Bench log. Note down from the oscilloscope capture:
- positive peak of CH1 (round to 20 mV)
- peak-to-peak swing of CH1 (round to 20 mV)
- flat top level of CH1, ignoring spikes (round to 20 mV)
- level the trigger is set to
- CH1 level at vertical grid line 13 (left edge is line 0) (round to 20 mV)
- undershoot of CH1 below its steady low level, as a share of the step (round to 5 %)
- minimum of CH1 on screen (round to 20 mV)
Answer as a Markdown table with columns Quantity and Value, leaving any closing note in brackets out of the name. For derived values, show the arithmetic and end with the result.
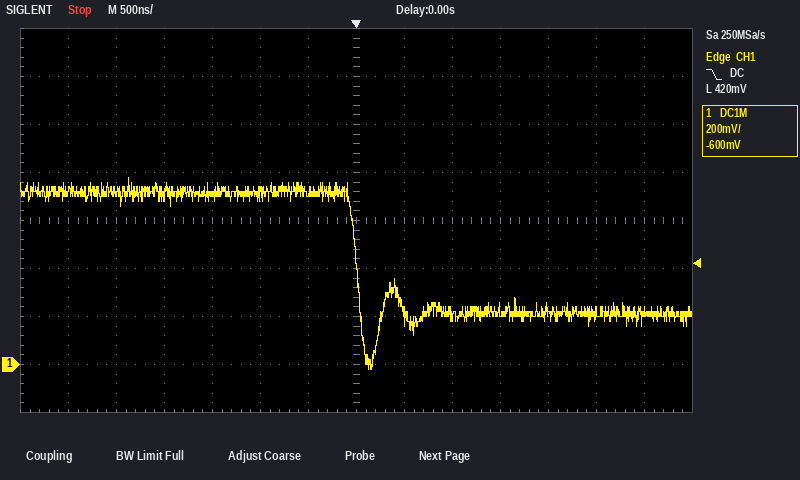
| Quantity | Value |
|---|---|
| positive peak of CH1 | 780 mV |
| peak-to-peak swing of CH1 | 780 mV − (-20 mV) = 800 mV |
| flat top level of CH1, ignoring spikes | 720 mV |
| level the trigger is set to | 420 mV |
| CH1 level at vertical grid line 13 (left edge is line 0) | 220 mV |
| undershoot of CH1 below its steady low level, as a share of the step | 45 % |
| minimum of CH1 on screen | -20 mV |
